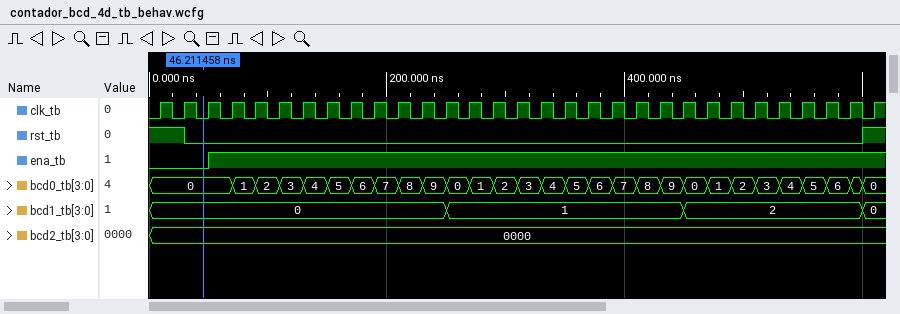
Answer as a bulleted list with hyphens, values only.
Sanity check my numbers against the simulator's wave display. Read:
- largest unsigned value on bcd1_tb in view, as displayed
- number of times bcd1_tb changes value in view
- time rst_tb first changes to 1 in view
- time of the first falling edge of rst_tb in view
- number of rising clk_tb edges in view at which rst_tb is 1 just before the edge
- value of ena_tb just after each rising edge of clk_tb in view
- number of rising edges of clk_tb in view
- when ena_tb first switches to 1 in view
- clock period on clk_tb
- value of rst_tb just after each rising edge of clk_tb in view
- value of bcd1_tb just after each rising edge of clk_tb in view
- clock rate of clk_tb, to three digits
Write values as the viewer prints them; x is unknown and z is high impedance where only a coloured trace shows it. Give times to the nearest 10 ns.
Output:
- 2
- 3
- 600 ns
- 30 ns
- 3
- 0 0 1 1 1 1 1 1 1 1 1 1 1 1 1 1 1 1 1 1 1 1 1 1 1 1 1 1 1 1 1
- 31
- 50 ns
- 20 ns
- 1 0 0 0 0 0 0 0 0 0 0 0 0 0 0 0 0 0 0 0 0 0 0 0 0 0 0 0 0 0 1
- 0, 0, 0, 0, 0, 0, 0, 0, 0, 0, 0, 0, 1, 1, 1, 1, 1, 1, 1, 1, 1, 1, 2, 2, 2, 2, 2, 2, 2, 2, 0
- 50.0 MHz
